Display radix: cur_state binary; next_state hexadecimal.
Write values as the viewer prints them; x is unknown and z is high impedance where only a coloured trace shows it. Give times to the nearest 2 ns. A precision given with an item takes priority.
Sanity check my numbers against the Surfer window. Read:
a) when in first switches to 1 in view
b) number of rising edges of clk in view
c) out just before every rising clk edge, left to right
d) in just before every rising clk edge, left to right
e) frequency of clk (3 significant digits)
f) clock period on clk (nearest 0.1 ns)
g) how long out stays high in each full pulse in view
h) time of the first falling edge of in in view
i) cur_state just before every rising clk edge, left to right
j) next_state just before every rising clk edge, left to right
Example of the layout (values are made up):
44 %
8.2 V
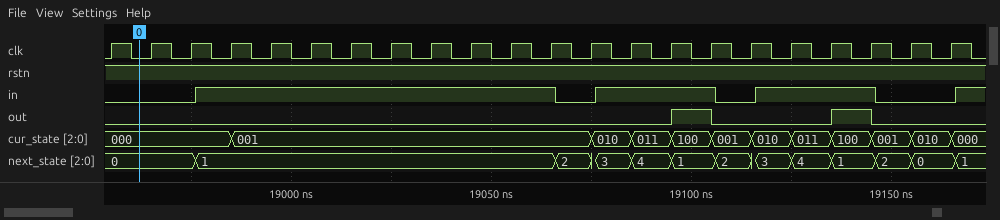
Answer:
18976 ns
22
0 0 0 0 0 0 0 0 0 0 0 0 0 0 0 1 0 0 0 1 0 0
0 0 0 1 1 1 1 1 1 1 1 1 0 1 1 1 0 1 1 1 0 0
100 MHz
10 ns
10 ns, 10 ns
19066 ns
000, 000, 000, 000, 001, 001, 001, 001, 001, 001, 001, 001, 001, 010, 011, 100, 001, 010, 011, 100, 001, 010
0, 0, 0, 1, 1, 1, 1, 1, 1, 1, 1, 1, 2, 3, 4, 1, 2, 3, 4, 1, 2, 0
